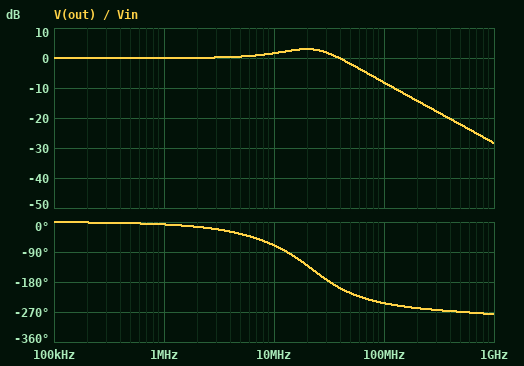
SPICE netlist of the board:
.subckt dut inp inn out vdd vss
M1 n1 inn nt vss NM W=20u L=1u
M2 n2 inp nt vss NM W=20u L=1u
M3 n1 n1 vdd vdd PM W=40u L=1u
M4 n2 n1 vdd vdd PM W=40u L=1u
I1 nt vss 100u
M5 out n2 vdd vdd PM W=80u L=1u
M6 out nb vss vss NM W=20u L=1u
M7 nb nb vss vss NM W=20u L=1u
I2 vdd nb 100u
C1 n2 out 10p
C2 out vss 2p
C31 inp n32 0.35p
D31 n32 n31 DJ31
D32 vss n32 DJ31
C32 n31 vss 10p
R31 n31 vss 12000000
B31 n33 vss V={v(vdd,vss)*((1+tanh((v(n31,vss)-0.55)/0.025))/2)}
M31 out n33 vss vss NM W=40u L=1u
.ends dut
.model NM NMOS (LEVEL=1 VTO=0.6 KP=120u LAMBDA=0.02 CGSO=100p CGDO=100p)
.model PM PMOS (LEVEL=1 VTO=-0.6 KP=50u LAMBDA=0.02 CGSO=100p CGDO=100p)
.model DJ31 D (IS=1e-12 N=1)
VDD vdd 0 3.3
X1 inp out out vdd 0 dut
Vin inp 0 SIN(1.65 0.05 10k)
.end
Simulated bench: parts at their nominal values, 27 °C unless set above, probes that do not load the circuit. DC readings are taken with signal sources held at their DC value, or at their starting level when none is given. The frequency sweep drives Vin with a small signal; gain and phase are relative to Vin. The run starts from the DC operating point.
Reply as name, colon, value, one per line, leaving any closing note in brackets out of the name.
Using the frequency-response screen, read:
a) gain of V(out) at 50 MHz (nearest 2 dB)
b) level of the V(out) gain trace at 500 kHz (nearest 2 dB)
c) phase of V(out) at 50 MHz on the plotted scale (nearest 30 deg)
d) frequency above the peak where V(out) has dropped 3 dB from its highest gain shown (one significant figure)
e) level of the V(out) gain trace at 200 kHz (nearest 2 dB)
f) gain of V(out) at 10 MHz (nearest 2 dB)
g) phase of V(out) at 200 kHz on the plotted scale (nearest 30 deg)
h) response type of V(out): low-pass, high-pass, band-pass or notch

gain of V(out) at 50 MHz: -2 dB
level of the V(out) gain trace at 500 kHz: 0 dB
phase of V(out) at 50 MHz on the plotted scale: -210 deg
frequency above the peak where V(out) has dropped 3 dB from its highest gain shown: 40 MHz
level of the V(out) gain trace at 200 kHz: 0 dB
gain of V(out) at 10 MHz: 2 dB
phase of V(out) at 200 kHz on the plotted scale: 0 deg
response type of V(out): low-pass, high-pass, band-pass or notch: low-pass
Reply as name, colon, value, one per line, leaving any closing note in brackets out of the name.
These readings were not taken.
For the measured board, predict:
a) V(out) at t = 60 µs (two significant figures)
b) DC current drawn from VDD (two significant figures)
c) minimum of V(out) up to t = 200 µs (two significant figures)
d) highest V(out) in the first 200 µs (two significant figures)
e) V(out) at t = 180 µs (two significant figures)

V(out) at t = 60 µs: 1.6 V
DC current drawn from VDD: 300 µA
minimum of V(out) up to t = 200 µs: 1.6 V
highest V(out) in the first 200 µs: 1.7 V
V(out) at t = 180 µs: 1.6 V
